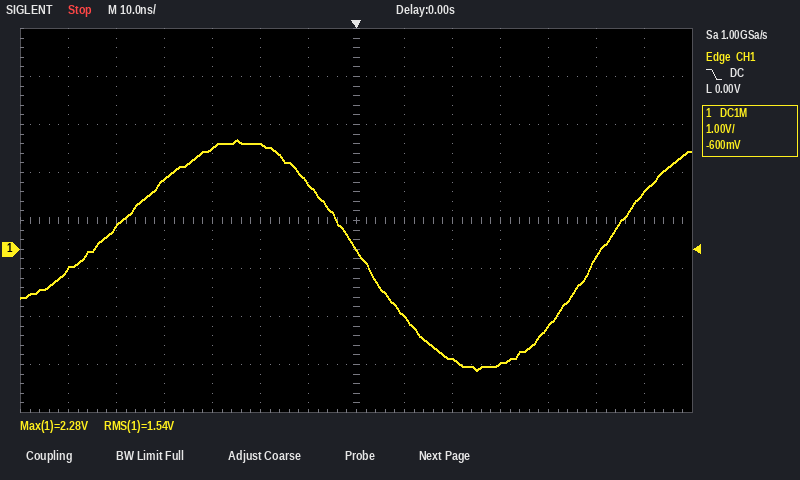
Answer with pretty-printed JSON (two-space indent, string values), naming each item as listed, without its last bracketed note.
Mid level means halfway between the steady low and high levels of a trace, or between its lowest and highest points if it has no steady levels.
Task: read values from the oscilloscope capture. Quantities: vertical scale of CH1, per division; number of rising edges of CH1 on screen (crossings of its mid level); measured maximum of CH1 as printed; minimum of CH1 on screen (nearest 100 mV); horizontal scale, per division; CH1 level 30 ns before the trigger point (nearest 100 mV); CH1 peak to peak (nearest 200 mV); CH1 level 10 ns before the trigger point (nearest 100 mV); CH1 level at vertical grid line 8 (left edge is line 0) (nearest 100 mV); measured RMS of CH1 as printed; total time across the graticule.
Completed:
{
  "vertical scale of CH1, per division": "1 V",
  "number of rising edges of CH1 on screen": "2",
  "measured maximum of CH1 as printed": "2.28 V",
  "minimum of CH1 on screen": "-2.5 V",
  "horizontal scale, per division": "10 ns",
  "CH1 level 30 ns before the trigger point": "2.1 V",
  "CH1 peak to peak": "4.8 V",
  "CH1 level 10 ns before the trigger point": "1.4 V",
  "CH1 level at vertical grid line 8 (left edge is line 0)": "-1.4 V",
  "measured RMS of CH1 as printed": "1.54 V",
  "total time across the graticule": "140 ns"
}
